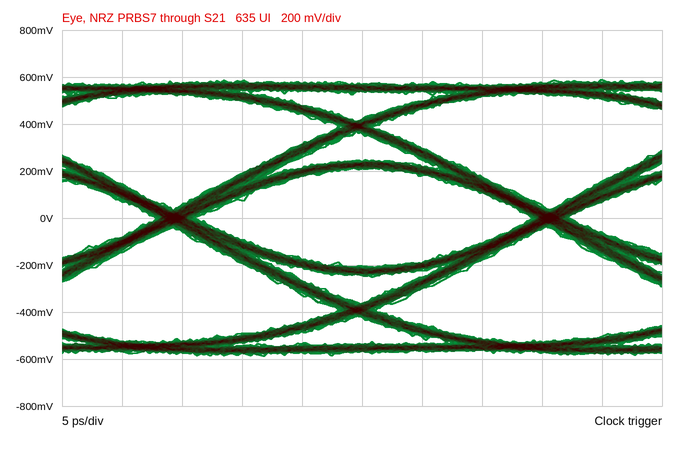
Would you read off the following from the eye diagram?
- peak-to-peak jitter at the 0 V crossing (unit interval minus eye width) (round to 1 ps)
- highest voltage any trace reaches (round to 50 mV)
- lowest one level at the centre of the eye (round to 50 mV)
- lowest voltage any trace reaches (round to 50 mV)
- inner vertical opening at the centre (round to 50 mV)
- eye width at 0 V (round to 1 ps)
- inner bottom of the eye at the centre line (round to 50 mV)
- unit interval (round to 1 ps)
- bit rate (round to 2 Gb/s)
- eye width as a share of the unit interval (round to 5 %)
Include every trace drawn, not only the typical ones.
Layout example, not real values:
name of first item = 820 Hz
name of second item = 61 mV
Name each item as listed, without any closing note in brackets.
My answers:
peak-to-peak jitter at the 0 V crossing (unit interval minus eye width) = 3 ps
highest voltage any trace reaches = 600 mV
lowest one level at the centre of the eye = 200 mV
lowest voltage any trace reaches = -600 mV
inner vertical opening at the centre = 400 mV
eye width at 0 V = 28 ps
inner bottom of the eye at the centre line = -200 mV
unit interval = 31 ps
bit rate = 32 Gb/s
eye width as a share of the unit interval = 90 %
